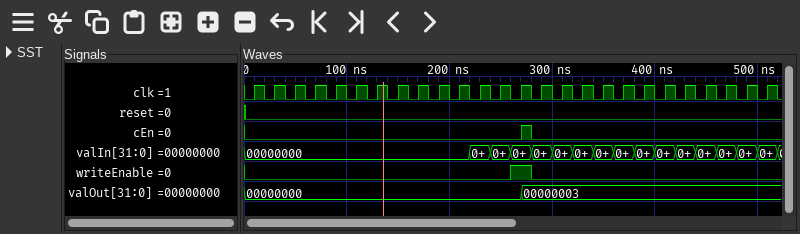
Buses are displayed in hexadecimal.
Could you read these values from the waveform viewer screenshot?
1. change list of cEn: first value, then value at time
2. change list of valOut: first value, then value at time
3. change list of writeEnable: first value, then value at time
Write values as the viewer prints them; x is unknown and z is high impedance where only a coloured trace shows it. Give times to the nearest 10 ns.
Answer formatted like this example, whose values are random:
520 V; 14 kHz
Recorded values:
0, 1 at 270 ns, 0 at 280 ns; 00000000, 00000003 at 270 ns; 0, 1 at 260 ns, 0 at 280 ns
